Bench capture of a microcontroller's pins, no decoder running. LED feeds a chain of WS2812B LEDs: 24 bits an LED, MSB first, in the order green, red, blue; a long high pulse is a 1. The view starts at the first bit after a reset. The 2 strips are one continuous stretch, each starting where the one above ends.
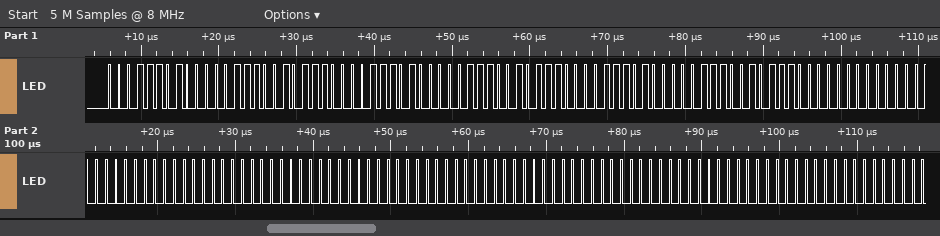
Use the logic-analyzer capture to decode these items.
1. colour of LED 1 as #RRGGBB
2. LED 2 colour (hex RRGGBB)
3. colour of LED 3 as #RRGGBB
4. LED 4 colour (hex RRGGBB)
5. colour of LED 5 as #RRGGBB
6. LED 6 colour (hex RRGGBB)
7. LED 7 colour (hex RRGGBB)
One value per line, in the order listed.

#071D2E
#071D2E
#071D2E
#000000
#000000
#000000
#000000
